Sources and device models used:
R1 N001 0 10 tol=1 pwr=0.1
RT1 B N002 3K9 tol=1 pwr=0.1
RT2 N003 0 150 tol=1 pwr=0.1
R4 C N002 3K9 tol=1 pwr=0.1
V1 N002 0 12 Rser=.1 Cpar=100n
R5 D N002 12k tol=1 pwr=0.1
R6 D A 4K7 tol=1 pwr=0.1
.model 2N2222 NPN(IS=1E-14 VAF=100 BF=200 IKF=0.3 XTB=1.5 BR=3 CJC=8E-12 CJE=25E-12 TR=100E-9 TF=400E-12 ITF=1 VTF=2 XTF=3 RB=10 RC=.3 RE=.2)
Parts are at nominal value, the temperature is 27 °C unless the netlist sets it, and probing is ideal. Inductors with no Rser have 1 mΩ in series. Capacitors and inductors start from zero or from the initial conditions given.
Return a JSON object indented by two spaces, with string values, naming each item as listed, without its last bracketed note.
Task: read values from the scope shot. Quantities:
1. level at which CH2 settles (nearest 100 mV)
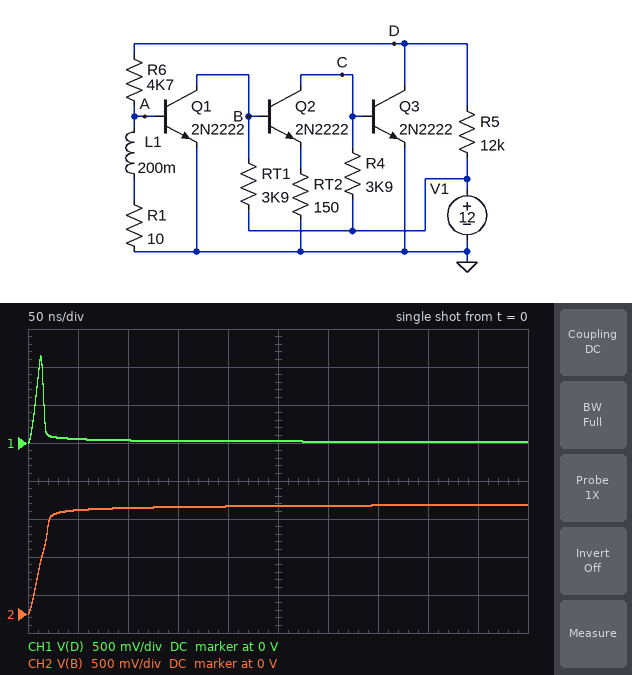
{
  "level at which CH2 settles": "1.4 V"
}
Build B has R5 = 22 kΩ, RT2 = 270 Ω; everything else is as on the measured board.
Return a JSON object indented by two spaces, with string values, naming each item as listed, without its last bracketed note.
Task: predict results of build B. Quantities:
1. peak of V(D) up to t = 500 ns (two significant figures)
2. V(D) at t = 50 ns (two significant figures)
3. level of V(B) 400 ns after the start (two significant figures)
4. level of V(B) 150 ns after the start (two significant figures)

{
  "peak of V(D) up to t = 500 ns": "880 mV",
  "V(D) at t = 50 ns": "43 mV",
  "level of V(B) 400 ns after the start": "1.5 V",
  "level of V(B) 150 ns after the start": "1.4 V"
}
